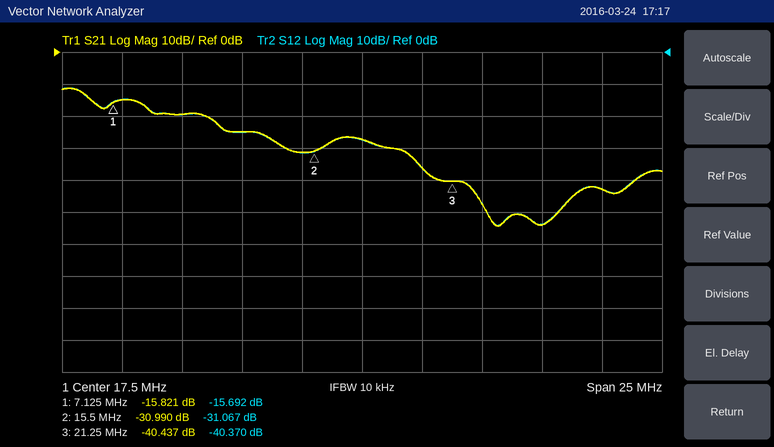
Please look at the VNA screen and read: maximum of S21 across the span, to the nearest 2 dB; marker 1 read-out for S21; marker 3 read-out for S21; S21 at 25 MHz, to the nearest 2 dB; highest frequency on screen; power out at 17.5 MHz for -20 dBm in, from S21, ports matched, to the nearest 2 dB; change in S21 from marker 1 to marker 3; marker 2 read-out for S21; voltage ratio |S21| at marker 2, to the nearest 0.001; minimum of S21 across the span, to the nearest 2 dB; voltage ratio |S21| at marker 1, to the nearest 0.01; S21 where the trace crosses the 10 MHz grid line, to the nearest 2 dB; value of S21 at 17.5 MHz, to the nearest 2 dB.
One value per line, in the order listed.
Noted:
-12 dB
-15.821 dB
-40.437 dB
-54 dB
30 MHz
-48 dBm
-24.616 dB
-30.990 dB
0.028
-54 dB
0.16
-20 dB
-28 dB
